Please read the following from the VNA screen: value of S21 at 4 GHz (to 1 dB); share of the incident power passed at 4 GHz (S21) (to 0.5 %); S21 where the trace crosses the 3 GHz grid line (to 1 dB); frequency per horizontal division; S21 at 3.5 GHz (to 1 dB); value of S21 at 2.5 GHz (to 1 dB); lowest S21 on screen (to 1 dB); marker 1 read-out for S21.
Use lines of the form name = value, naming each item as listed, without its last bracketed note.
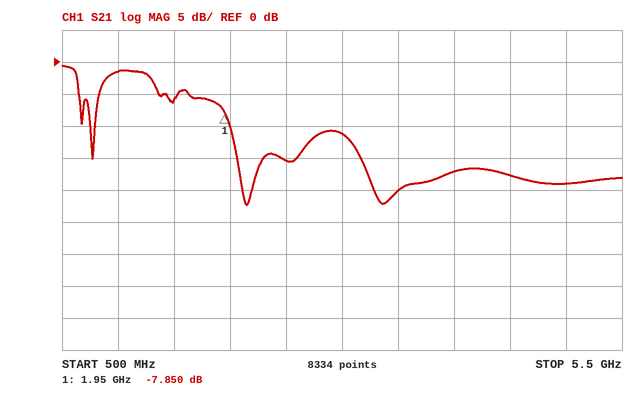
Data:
value of S21 at 4 GHz = -17 dB
share of the incident power passed at 4 GHz (S21) = 2.0 %
S21 where the trace crosses the 3 GHz grid line = -11 dB
frequency per horizontal division = 500 MHz
S21 at 3.5 GHz = -20 dB
value of S21 at 2.5 GHz = -15 dB
lowest S21 on screen = -22 dB
marker 1 read-out for S21 = -7.850 dB
